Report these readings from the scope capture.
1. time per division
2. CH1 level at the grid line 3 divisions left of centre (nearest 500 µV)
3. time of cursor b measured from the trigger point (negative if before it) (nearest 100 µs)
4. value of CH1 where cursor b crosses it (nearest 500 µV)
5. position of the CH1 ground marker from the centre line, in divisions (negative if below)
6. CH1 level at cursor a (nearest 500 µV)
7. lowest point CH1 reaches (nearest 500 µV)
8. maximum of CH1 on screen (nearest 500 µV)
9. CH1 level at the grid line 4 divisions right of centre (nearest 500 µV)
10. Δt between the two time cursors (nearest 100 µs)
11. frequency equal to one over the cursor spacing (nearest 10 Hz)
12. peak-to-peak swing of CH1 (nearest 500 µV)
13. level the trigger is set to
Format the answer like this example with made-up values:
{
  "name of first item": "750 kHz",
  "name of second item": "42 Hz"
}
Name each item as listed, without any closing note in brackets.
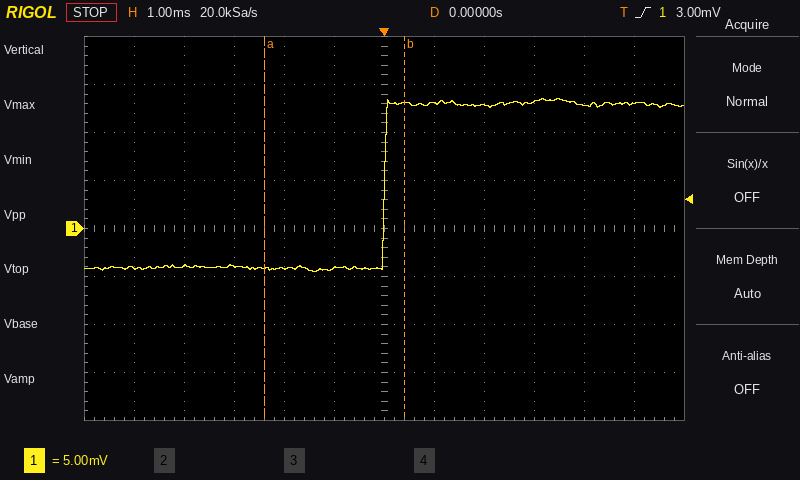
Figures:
{
  "time per division": "1 ms",
  "CH1 level at the grid line 3 divisions left of centre": "-4.0 mV",
  "time of cursor b measured from the trigger point (negative if before it)": "+400 µs",
  "value of CH1 where cursor b crosses it": "13.0 mV",
  "position of the CH1 ground marker from the centre line, in divisions": "0.0 div",
  "CH1 level at cursor a": "-4.0 mV",
  "lowest point CH1 reaches": "-4.5 mV",
  "maximum of CH1 on screen": "13.5 mV",
  "CH1 level at the grid line 4 divisions right of centre": "13.0 mV",
  "Δt between the two time cursors": "2.8 ms",
  "frequency equal to one over the cursor spacing": "360 Hz",
  "peak-to-peak swing of CH1": "18.0 mV",
  "level the trigger is set to": "3.00 mV"
}
